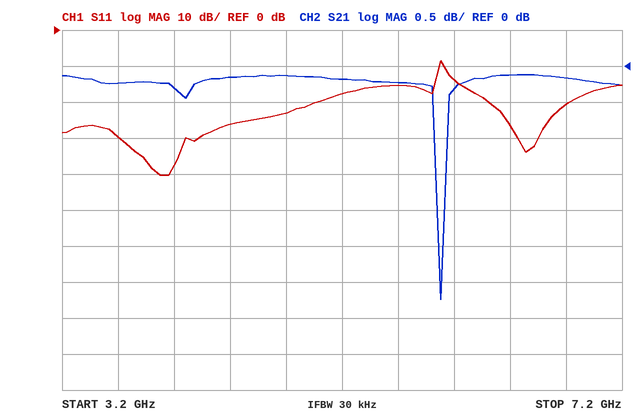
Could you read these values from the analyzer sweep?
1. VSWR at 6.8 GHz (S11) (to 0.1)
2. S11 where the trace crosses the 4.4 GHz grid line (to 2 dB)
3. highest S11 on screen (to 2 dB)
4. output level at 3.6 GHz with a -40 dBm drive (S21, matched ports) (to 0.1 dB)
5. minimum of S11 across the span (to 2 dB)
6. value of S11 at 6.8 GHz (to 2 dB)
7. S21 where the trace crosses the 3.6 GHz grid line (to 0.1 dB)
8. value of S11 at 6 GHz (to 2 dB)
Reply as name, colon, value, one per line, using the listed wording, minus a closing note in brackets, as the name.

VSWR at 6.8 GHz (S11): 1.2
S11 where the trace crosses the 4.4 GHz grid line: -26 dB
highest S11 on screen: -8 dB
output level at 3.6 GHz with a -40 dBm drive (S21, matched ports): -40.2 dBm
minimum of S11 across the span: -40 dB
value of S11 at 6.8 GHz: -20 dB
S21 where the trace crosses the 3.6 GHz grid line: -0.2 dB
value of S11 at 6 GHz: -14 dB
